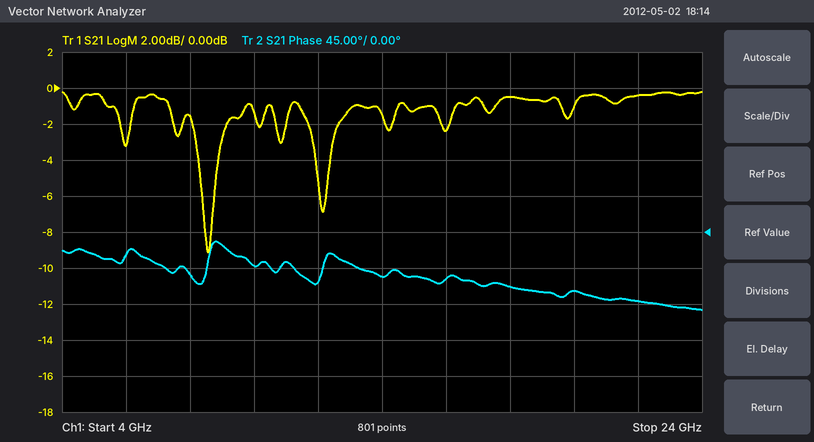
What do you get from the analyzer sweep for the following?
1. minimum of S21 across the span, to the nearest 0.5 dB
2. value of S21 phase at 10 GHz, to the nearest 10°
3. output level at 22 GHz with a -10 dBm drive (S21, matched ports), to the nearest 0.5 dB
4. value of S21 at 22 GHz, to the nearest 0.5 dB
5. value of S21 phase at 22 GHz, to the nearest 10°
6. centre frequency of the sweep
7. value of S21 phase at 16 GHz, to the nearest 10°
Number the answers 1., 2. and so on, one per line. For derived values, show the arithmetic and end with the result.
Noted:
1. -9.0 dB
2. -40°
3. -10 dBm + (-0.5 dB) = -10.5 dBm
4. -0.5 dB
5. -90°
6. 14 GHz
7. -60°
